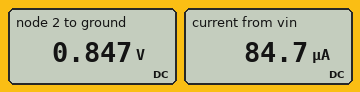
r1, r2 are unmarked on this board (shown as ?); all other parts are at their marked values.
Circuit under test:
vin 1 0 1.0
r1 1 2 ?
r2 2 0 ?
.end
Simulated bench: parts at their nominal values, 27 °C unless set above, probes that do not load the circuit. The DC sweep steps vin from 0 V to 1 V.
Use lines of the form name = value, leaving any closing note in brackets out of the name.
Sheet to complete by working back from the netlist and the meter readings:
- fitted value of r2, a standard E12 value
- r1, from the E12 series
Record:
fitted value of r2, a standard E12 value = 10 kΩ
r1, from the E12 series = 1.8 kΩ
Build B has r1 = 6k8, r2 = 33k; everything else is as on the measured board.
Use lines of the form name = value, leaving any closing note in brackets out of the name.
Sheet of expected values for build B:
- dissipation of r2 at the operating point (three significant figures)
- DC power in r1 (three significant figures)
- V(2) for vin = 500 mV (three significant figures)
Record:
dissipation of r2 at the operating point = 20.8 µW
DC power in r1 = 4.29 µW
V(2) for vin = 500 mV = 415 mV
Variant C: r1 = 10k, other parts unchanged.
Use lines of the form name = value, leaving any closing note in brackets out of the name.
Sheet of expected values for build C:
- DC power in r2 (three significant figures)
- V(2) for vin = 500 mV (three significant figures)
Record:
DC power in r2 = 25.0 µW
V(2) for vin = 500 mV = 250 mV
